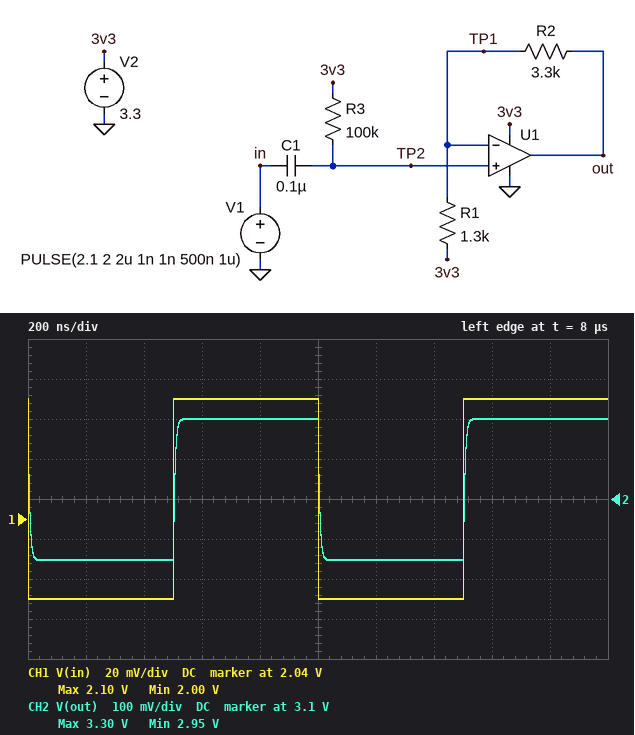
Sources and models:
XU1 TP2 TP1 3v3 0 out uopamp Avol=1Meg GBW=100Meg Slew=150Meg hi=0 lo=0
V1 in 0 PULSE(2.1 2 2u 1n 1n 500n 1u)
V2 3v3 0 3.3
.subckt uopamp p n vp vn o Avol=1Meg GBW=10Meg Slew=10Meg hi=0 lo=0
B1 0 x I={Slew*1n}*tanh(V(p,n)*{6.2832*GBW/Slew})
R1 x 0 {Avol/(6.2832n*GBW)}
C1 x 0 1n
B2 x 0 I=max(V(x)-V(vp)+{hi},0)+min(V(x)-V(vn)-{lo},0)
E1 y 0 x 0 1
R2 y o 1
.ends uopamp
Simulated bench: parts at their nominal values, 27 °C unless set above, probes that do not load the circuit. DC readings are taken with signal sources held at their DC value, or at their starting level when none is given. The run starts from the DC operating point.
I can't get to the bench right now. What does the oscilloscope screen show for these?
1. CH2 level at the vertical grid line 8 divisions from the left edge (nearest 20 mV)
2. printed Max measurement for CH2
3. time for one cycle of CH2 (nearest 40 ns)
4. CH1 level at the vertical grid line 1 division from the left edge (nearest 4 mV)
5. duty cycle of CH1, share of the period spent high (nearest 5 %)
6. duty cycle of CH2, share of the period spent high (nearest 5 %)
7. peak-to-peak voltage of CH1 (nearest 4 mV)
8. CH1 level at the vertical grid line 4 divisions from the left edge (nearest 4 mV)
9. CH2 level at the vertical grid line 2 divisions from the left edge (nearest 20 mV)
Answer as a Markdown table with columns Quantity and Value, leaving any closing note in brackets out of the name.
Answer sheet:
| Quantity | Value |
|---|---|
| CH2 level at the vertical grid line 8 divisions from the left edge | 3.30 V |
| printed Max measurement for CH2 | 3.30 V |
| time for one cycle of CH2 | 1.00 µs |
| CH1 level at the vertical grid line 1 division from the left edge | 2.000 V |
| duty cycle of CH1, share of the period spent high | 50 % |
| duty cycle of CH2, share of the period spent high | 50 % |
| peak-to-peak voltage of CH1 | 100 mV |
| CH1 level at the vertical grid line 4 divisions from the left edge | 2.100 V |
| CH2 level at the vertical grid line 2 divisions from the left edge | 2.94 V |
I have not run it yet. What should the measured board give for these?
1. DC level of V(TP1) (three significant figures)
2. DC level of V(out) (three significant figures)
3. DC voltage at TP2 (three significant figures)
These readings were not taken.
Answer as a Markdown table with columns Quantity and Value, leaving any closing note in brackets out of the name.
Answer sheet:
| Quantity | Value |
|---|---|
| DC level of V(TP1) | 3.30 V |
| DC level of V(out) | 3.30 V |
| DC voltage at TP2 | 3.30 V |
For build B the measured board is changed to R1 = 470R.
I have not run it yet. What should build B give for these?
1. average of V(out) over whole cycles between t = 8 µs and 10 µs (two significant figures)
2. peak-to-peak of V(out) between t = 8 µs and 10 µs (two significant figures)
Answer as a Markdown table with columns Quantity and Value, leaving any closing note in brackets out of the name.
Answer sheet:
| Quantity | Value |
|---|---|
| average of V(out) over whole cycles between t = 8 µs and 10 µs | 2.9 V |
| peak-to-peak of V(out) between t = 8 µs and 10 µs | 800 mV |
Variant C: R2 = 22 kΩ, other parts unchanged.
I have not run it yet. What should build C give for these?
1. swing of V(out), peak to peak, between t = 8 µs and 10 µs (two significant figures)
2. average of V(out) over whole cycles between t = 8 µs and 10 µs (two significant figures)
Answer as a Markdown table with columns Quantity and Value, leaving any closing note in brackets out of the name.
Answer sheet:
| Quantity | Value |
|---|---|
| swing of V(out), peak to peak, between t = 8 µs and 10 µs | 1.8 V |
| average of V(out) over whole cycles between t = 8 µs and 10 µs | 2.4 V |
